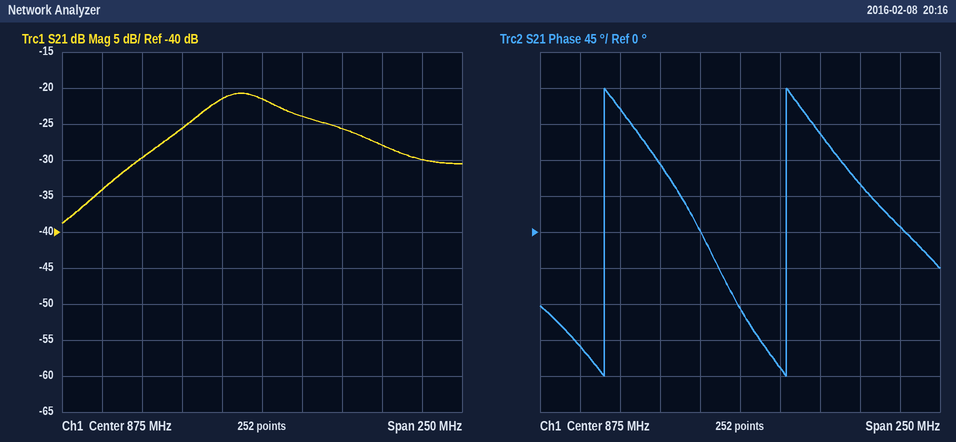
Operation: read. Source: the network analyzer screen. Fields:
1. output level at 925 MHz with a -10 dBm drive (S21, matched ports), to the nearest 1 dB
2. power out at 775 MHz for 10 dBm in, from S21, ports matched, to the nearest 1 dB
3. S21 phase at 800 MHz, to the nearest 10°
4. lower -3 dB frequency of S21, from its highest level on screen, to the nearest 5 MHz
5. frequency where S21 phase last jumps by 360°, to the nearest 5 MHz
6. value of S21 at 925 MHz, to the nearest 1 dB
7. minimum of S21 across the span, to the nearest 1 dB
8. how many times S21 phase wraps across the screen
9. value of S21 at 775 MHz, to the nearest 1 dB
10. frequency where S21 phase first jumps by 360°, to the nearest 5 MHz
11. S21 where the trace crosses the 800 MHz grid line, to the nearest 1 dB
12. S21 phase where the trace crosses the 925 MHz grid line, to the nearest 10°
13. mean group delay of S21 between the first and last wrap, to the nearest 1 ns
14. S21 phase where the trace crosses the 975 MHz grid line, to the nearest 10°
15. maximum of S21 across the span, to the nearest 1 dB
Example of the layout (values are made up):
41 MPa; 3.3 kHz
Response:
-36 dBm; -24 dBm; 150°; 835 MHz; 905 MHz; -26 dB; -39 dB; 2; -34 dB; 790 MHz; -30 dB; 120°; 9 ns; 10°; -21 dB
